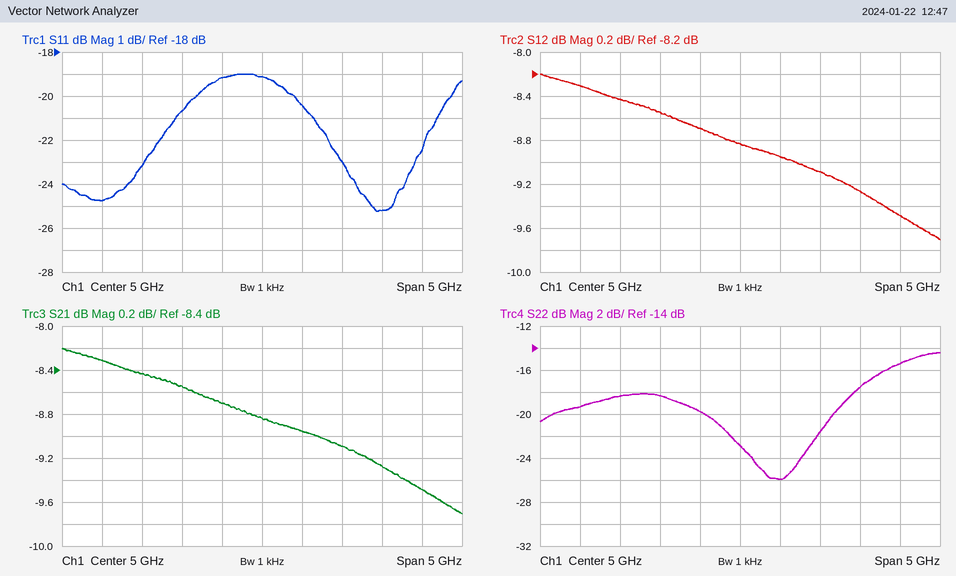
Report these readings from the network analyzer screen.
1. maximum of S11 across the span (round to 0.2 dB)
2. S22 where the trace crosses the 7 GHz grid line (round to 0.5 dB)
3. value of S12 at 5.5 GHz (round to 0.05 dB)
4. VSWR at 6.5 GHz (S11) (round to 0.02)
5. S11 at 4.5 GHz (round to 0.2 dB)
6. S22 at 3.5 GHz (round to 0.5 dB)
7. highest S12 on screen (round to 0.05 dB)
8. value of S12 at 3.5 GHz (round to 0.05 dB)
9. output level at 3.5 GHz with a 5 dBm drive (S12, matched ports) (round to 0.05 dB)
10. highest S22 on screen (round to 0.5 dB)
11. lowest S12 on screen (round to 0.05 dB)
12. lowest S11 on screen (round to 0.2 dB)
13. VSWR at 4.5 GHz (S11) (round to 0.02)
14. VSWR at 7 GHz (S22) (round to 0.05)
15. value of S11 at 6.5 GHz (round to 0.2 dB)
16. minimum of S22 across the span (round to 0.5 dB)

-19.0 dB
-15.5 dB
-8.95 dB
1.12
-19.2 dB
-18.5 dB
-8.20 dB
-8.45 dB
-3.45 dBm
-14.5 dB
-9.70 dB
-25.2 dB
1.24
1.40
-25.2 dB
-26.0 dB
